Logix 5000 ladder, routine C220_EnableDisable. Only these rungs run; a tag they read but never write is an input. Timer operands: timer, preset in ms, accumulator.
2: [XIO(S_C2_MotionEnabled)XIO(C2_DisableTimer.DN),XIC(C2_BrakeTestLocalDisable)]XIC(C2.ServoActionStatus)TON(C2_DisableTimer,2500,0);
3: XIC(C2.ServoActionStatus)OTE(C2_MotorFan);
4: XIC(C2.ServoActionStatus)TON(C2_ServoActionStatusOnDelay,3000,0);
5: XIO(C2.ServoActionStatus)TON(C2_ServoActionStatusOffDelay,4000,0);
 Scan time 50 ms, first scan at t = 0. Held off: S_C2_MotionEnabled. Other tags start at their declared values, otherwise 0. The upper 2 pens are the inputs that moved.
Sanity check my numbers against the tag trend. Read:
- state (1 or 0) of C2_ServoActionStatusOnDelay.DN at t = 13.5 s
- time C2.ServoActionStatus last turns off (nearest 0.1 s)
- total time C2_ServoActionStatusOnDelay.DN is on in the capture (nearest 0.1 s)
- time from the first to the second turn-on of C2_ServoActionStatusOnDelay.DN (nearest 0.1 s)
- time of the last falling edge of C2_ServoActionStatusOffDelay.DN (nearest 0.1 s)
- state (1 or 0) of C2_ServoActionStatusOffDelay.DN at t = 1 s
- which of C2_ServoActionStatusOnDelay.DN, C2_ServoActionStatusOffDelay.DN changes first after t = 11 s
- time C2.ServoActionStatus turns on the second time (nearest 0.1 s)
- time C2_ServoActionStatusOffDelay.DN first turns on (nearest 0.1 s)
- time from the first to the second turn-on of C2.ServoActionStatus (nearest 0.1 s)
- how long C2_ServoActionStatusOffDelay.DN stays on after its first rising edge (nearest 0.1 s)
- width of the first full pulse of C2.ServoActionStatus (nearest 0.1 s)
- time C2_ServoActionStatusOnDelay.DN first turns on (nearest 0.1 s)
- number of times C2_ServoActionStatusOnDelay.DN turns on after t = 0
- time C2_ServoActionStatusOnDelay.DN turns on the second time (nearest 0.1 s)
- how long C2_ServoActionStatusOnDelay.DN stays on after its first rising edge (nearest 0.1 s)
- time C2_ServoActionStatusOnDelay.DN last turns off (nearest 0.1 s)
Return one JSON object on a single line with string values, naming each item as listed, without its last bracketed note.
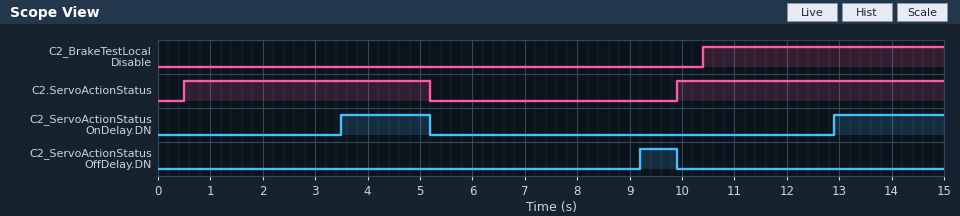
{"state (1 or 0) of C2_ServoActionStatusOnDelay.DN at t = 13.5 s": "1", "time C2.ServoActionStatus last turns off": "5.2 s", "total time C2_ServoActionStatusOnDelay.DN is on in the capture": "3.8 s", "time from the first to the second turn-on of C2_ServoActionStatusOnDelay.DN": "9.4 s", "time of the last falling edge of C2_ServoActionStatusOffDelay.DN": "9.9 s", "state (1 or 0) of C2_ServoActionStatusOffDelay.DN at t = 1 s": "0", "which of C2_ServoActionStatusOnDelay.DN, C2_ServoActionStatusOffDelay.DN changes first after t = 11 s": "C2_ServoActionStatusOnDelay.DN", "time C2.ServoActionStatus turns on the second time": "9.9 s", "time C2_ServoActionStatusOffDelay.DN first turns on": "9.2 s", "time from the first to the second turn-on of C2.ServoActionStatus": "9.4 s", "how long C2_ServoActionStatusOffDelay.DN stays on after its first rising edge": "0.7 s", "width of the first full pulse of C2.ServoActionStatus": "4.7 s", "time C2_ServoActionStatusOnDelay.DN first turns on": "3.5 s", "number of times C2_ServoActionStatusOnDelay.DN turns on after t = 0": "2", "time C2_ServoActionStatusOnDelay.DN turns on the second time": "12.9 s", "how long C2_ServoActionStatusOnDelay.DN stays on after its first rising edge": "1.7 s", "time C2_ServoActionStatusOnDelay.DN last turns off": "5.2 s"}
